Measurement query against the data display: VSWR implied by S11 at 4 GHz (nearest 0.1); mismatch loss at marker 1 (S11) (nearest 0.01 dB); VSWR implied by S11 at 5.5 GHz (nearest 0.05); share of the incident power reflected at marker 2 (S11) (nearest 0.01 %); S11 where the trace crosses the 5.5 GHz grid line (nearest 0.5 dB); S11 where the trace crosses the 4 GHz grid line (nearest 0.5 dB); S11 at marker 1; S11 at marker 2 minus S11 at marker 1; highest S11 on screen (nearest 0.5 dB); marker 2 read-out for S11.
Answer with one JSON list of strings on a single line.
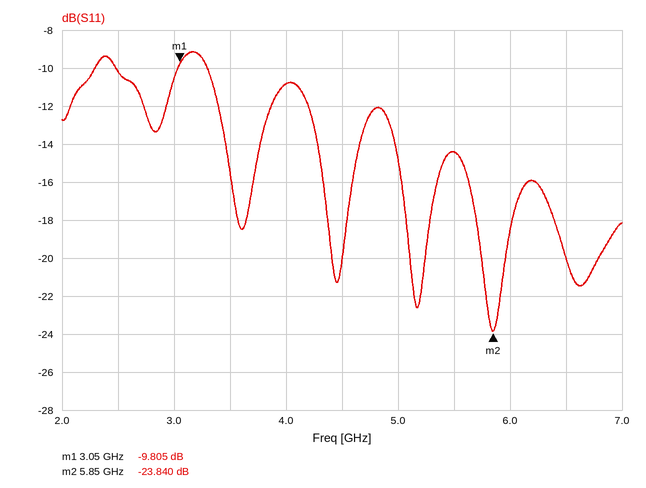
["1.8", "0.48 dB", "1.45", "0.41 %", "-14.5 dB", "-11.0 dB", "-9.805 dB", "-14.035 dB", "-9.0 dB", "-23.840 dB"]
